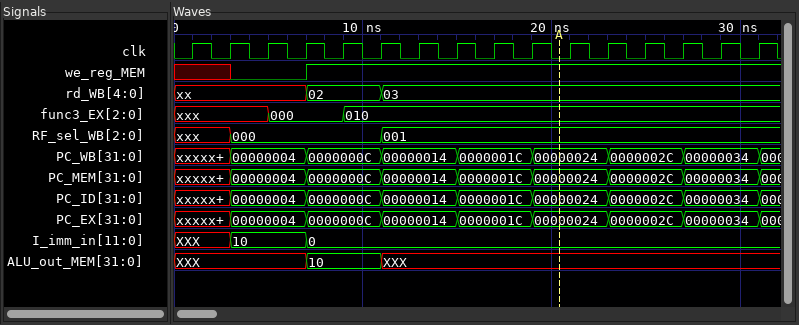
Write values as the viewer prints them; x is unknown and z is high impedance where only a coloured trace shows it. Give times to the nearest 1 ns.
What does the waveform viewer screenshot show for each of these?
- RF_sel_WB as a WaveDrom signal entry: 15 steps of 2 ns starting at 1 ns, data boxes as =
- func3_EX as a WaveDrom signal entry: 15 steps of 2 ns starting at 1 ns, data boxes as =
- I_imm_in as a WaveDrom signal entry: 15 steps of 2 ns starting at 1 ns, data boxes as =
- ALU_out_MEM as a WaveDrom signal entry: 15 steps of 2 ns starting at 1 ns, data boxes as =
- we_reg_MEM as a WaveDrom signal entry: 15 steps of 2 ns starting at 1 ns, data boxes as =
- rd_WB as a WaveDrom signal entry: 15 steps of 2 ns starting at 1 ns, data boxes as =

{name: 'RF_sel_WB', wave: 'x=...=.........', data: '000 001'}
{name: 'func3_EX', wave: 'x.=.=..........', data: '000 010'}
{name: 'I_imm_in', wave: 'x=.=...........', data: '10 0'}
{name: 'ALU_out_MEM', wave: 'x..=.x.........', data: '10'}
{name: 'we_reg_MEM', wave: 'x0.1...........'}
{name: 'rd_WB', wave: 'x..=.=.........', data: '02 03'}
